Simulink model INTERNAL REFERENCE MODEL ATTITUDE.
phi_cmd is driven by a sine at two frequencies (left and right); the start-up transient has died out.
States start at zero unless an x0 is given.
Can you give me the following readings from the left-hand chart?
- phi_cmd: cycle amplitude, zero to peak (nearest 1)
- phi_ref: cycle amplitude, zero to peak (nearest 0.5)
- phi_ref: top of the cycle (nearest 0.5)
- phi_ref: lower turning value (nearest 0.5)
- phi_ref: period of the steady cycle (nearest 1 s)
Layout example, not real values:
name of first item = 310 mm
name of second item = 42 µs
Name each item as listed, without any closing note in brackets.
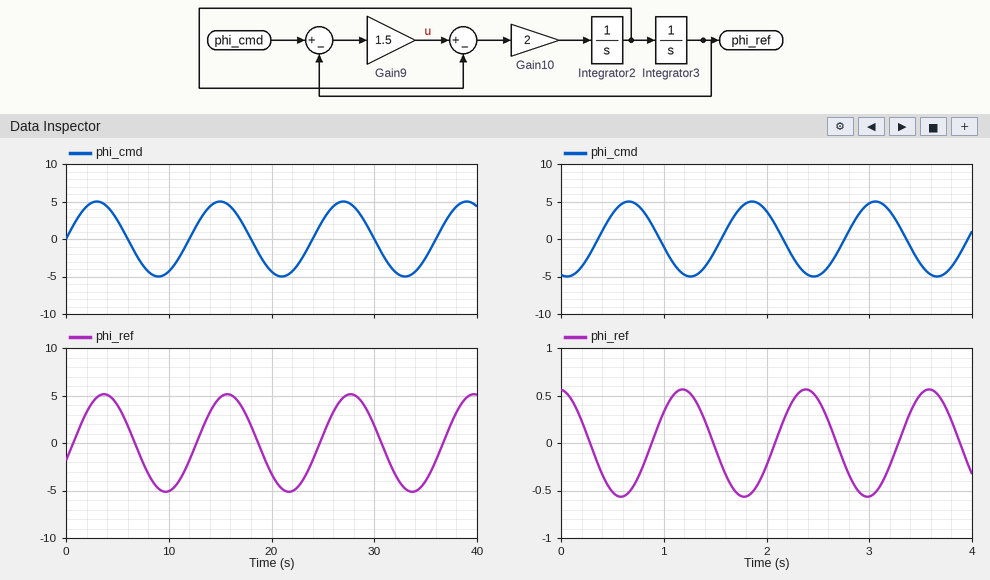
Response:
phi_cmd: cycle amplitude, zero to peak = 5
phi_ref: cycle amplitude, zero to peak = 5.0
phi_ref: top of the cycle = 5.0
phi_ref: lower turning value = -5.0
phi_ref: period of the steady cycle = 12 s
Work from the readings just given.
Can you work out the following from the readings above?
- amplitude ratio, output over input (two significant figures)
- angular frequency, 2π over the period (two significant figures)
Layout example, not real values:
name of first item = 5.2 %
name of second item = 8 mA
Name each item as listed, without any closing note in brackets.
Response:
amplitude ratio, output over input = 1.0
angular frequency, 2π over the period = 0.52 rad/s
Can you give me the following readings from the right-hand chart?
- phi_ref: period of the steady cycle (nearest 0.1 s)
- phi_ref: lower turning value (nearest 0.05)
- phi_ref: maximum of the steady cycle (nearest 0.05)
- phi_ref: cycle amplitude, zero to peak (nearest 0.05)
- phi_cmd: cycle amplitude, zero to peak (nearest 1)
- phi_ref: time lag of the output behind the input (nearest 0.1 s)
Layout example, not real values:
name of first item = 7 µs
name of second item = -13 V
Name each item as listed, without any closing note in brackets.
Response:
phi_ref: period of the steady cycle = 1.2 s
phi_ref: lower turning value = -0.55
phi_ref: maximum of the steady cycle = 0.55
phi_ref: cycle amplitude, zero to peak = 0.55
phi_cmd: cycle amplitude, zero to peak = 5
phi_ref: time lag of the output behind the input = 0.5 s
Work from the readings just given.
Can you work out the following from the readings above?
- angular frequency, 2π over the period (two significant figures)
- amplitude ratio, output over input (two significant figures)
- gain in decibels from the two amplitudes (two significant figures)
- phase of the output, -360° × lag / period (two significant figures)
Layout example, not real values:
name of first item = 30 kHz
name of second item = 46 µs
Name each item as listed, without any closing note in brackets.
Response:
angular frequency, 2π over the period = 5.2 rad/s
amplitude ratio, output over input = 0.11
gain in decibels from the two amplitudes = -19 dB
phase of the output, -360° × lag / period = -150°
